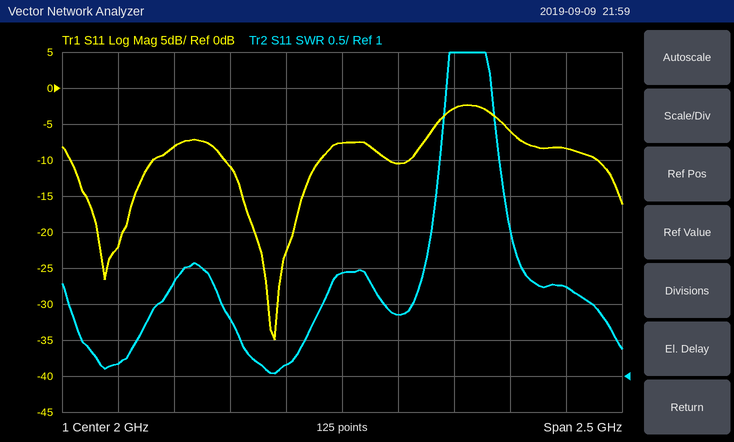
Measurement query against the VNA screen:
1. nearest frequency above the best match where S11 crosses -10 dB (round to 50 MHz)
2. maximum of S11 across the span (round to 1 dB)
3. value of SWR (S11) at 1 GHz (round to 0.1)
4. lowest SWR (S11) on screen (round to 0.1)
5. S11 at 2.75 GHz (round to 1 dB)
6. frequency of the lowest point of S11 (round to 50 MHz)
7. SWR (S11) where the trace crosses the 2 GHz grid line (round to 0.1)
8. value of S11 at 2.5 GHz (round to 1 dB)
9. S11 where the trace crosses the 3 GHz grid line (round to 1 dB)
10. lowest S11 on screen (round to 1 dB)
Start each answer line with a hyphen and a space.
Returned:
- 1.90 GHz
- -2 dB
- 1.2
- 1.0
- -6 dB
- 1.70 GHz
- 2.4
- -3 dB
- -8 dB
- -35 dB
